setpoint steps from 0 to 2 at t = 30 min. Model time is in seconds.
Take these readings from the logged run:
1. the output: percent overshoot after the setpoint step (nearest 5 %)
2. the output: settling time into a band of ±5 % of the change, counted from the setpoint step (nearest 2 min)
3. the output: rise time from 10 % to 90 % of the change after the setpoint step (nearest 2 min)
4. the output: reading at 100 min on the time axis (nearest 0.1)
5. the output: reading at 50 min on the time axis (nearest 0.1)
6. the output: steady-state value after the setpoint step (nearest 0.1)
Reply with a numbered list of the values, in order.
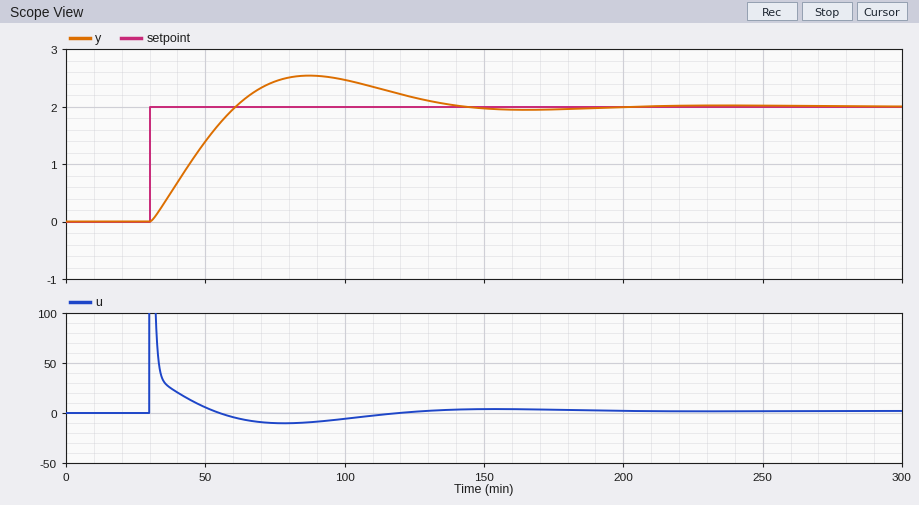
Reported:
1. 25 %
2. 100 min
3. 24 min
4. 2.5
5. 1.4
6. 2.0
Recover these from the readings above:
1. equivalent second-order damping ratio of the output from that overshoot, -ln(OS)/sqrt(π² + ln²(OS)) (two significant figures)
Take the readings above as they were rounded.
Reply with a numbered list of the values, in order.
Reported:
1. 0.40
